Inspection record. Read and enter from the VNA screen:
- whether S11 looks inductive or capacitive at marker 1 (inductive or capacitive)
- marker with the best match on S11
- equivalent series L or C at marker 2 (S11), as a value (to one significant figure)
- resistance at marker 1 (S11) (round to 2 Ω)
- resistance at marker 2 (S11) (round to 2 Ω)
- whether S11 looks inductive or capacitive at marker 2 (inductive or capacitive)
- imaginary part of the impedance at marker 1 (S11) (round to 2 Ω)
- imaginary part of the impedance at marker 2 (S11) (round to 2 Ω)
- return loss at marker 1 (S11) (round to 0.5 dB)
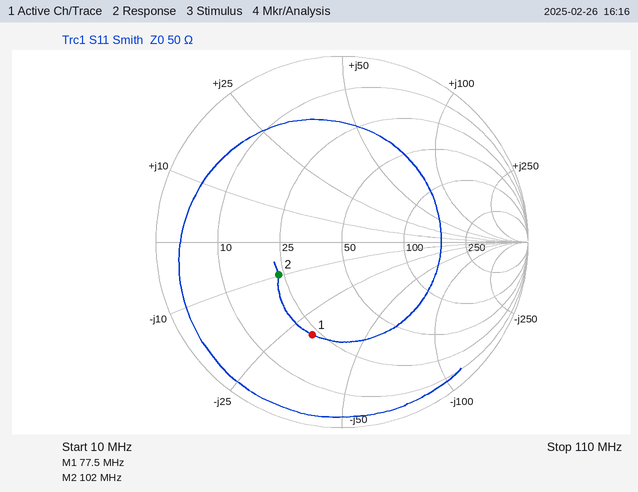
capacitive
marker 2
200 pF
22 Ω
24 Ω
capacitive
-32 Ω
-10 Ω
5.5 dB
